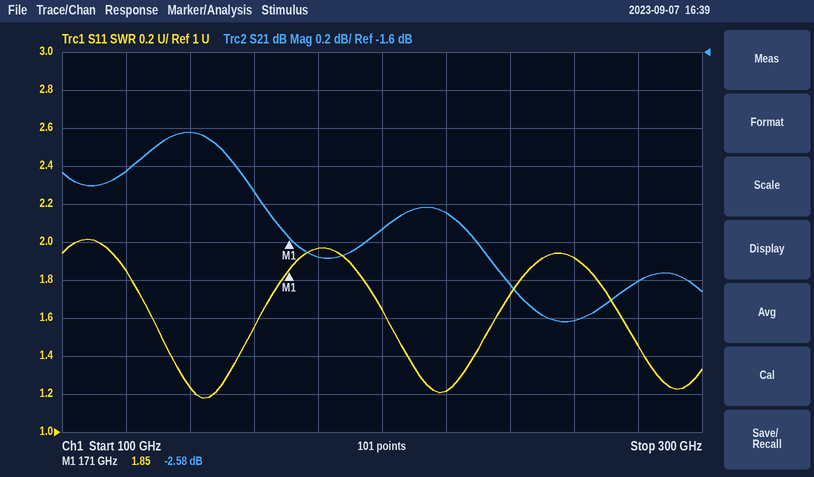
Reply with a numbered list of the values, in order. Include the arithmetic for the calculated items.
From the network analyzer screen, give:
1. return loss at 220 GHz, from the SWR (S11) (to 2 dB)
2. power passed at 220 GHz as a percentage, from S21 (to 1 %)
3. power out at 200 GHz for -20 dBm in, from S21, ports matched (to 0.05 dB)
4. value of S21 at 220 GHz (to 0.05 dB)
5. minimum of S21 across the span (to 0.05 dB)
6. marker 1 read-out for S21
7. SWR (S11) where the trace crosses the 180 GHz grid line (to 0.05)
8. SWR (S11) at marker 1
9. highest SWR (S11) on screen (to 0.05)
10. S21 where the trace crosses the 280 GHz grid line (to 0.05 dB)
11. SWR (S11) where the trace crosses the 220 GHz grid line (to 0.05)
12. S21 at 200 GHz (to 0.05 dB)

1. −20 log10((1.2 − 1)/(1.2 + 1)) ≈ 20.8 dB, so 20 dB to the nearest 2 dB
2. 10^(-2.45/10) ≈ 57 %
3. -20 dBm + (-2.55 dB) = -22.55 dBm
4. -2.45 dB
5. -3.00 dB
6. -2.58 dB
7. 1.95
8. 1.85
9. 2.00
10. -2.80 dB
11. 1.20
12. -2.55 dB
